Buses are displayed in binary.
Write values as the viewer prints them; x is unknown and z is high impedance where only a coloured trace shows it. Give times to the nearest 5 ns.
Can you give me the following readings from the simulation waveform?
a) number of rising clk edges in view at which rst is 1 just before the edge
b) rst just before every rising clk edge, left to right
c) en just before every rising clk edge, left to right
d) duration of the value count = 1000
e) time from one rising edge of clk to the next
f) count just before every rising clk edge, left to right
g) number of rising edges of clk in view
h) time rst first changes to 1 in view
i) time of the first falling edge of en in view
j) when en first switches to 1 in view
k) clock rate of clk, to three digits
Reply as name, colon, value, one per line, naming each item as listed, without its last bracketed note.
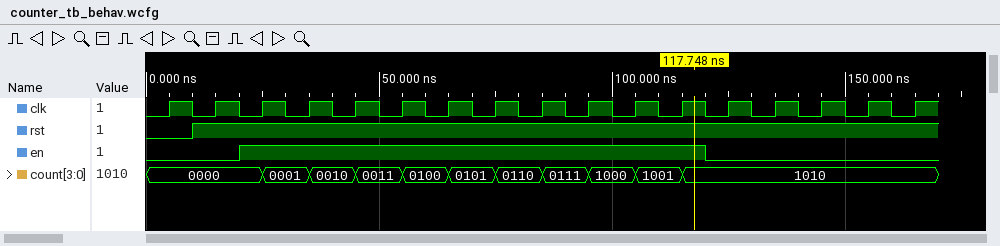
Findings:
number of rising clk edges in view at which rst is 1 just before the edge: 16
rst just before every rising clk edge, left to right: 0 1 1 1 1 1 1 1 1 1 1 1 1 1 1 1 1
en just before every rising clk edge, left to right: 0 0 1 1 1 1 1 1 1 1 1 1 0 0 0 0 0
duration of the value count = 1000: 10 ns
time from one rising edge of clk to the next: 10 ns
count just before every rising clk edge, left to right: 0000, 0000, 0000, 0001, 0010, 0011, 0100, 0101, 0110, 0111, 1000, 1001, 1010, 1010, 1010, 1010, 1010
number of rising edges of clk in view: 17
time rst first changes to 1 in view: 10 ns
time of the first falling edge of en in view: 120 ns
when en first switches to 1 in view: 20 ns
clock rate of clk, to three digits: 100 MHz
